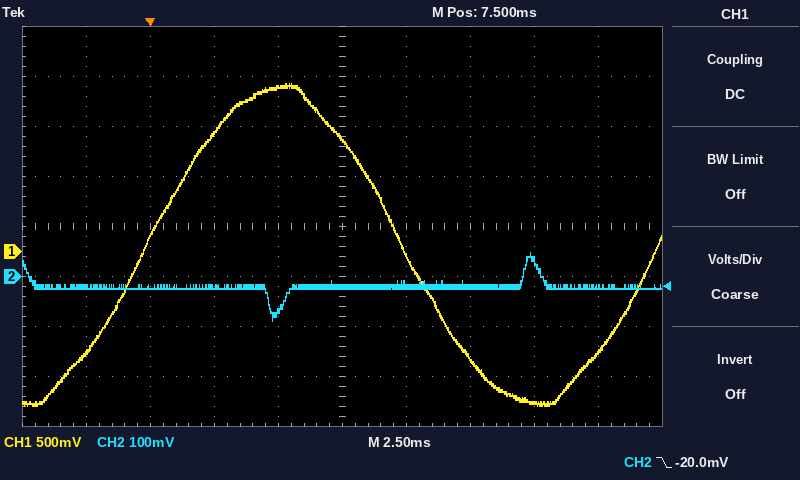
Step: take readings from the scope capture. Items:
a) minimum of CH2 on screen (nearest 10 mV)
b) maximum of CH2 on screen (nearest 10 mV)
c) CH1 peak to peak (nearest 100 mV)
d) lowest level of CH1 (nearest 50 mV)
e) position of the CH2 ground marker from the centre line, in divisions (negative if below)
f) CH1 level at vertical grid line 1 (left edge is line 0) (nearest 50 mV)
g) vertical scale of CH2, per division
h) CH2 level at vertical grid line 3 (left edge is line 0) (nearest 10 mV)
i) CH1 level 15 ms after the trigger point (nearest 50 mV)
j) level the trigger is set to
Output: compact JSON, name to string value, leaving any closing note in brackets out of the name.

{"minimum of CH2 on screen": "-90 mV", "maximum of CH2 on screen": "50 mV", "CH1 peak to peak": "3.20 V", "lowest level of CH1": "-1.55 V", "position of the CH2 ground marker from the centre line, in divisions": "-1.0 div", "CH1 level at vertical grid line 1 (left edge is line 0)": "-1.00 V", "vertical scale of CH2, per division": "100 mV", "CH2 level at vertical grid line 3 (left edge is line 0)": "-20 mV", "CH1 level 15 ms after the trigger point": "-1.50 V", "level the trigger is set to": "-20.0 mV"}
